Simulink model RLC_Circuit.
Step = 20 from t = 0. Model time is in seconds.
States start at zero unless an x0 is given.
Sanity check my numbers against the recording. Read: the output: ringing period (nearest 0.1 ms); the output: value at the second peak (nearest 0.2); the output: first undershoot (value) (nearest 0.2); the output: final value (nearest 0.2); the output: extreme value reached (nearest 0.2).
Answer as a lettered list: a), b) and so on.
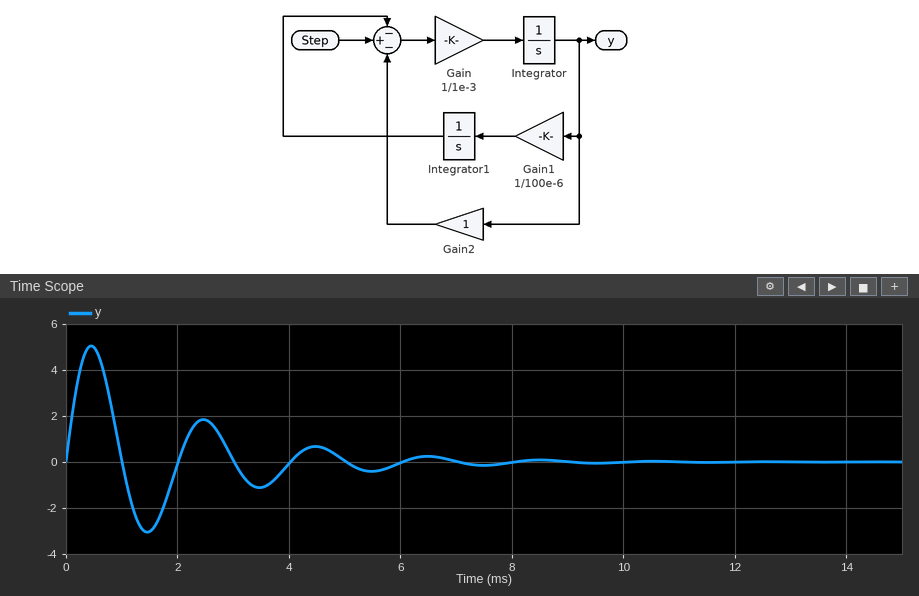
a) 2.0 ms
b) 1.8
c) -3.0
d) 0.0
e) 5.0
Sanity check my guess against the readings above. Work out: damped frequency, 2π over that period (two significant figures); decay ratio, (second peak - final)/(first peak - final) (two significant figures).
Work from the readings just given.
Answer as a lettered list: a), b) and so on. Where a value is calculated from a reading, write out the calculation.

a) 2π / 2 = 3.1 rad/ms
b) (1.8 - 0) / (5 - 0) = 0.36
